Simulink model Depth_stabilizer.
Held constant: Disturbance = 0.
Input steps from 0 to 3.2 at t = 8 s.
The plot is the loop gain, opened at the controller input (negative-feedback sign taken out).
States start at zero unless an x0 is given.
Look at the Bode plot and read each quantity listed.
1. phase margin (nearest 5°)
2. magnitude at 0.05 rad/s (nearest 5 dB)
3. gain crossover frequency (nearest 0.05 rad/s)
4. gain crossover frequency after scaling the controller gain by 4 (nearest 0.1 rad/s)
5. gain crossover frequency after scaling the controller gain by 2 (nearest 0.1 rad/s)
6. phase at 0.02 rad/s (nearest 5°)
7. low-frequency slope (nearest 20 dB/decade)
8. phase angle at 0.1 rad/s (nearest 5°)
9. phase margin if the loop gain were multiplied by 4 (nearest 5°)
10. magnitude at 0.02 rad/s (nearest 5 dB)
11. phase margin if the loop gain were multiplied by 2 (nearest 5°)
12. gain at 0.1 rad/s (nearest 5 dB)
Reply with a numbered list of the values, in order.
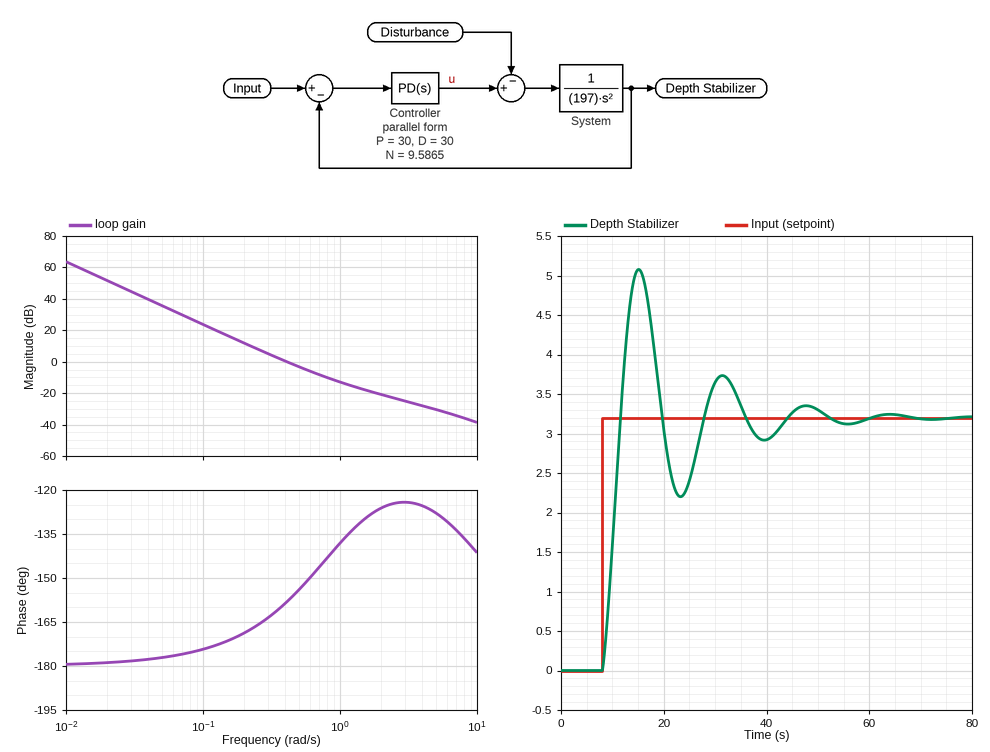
1. 20°
2. 35 dB
3. 0.40 rad/s
4. 0.9 rad/s
5. 0.6 rad/s
6. -180°
7. -40 dB/decade
8. -175°
9. 40°
10. 50 dB
11. 30°
12. 25 dB
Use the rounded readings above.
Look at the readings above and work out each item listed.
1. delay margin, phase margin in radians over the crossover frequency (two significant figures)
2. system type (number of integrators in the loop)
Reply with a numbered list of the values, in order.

1. 0.87 s
2. 2
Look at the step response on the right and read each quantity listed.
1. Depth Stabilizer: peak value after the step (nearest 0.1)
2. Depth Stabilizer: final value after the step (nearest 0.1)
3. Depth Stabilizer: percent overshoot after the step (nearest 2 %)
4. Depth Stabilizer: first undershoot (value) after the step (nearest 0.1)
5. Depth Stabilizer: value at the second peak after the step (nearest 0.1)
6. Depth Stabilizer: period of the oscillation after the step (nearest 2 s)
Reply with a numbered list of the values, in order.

1. 5.1
2. 3.2
3. 58 %
4. 2.2
5. 3.7
6. 16 s
